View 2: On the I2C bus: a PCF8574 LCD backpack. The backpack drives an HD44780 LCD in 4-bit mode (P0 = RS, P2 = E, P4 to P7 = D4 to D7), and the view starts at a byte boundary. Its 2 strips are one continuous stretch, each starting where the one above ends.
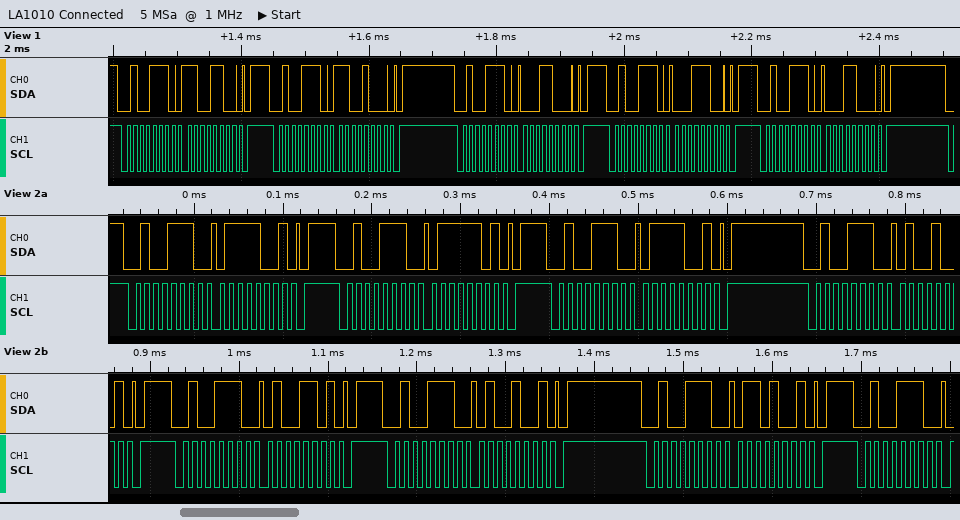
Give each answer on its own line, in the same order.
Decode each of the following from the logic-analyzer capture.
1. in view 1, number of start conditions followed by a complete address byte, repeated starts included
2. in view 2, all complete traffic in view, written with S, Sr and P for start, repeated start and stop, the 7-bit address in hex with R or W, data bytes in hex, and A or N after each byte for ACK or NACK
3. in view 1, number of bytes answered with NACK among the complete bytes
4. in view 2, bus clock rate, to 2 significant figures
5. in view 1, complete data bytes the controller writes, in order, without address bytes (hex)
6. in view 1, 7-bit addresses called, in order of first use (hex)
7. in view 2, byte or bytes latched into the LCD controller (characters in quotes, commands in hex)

5
S 27W A 79 A P S 27W A 7D A P S 27W A 79 A P S 27W A 49 A P S 27W A 4D A P S 27W A 49 A P S 27W A 69 A P S 27W A
0
100 kHz
CC C8 18 1C 18
0x27
't'
